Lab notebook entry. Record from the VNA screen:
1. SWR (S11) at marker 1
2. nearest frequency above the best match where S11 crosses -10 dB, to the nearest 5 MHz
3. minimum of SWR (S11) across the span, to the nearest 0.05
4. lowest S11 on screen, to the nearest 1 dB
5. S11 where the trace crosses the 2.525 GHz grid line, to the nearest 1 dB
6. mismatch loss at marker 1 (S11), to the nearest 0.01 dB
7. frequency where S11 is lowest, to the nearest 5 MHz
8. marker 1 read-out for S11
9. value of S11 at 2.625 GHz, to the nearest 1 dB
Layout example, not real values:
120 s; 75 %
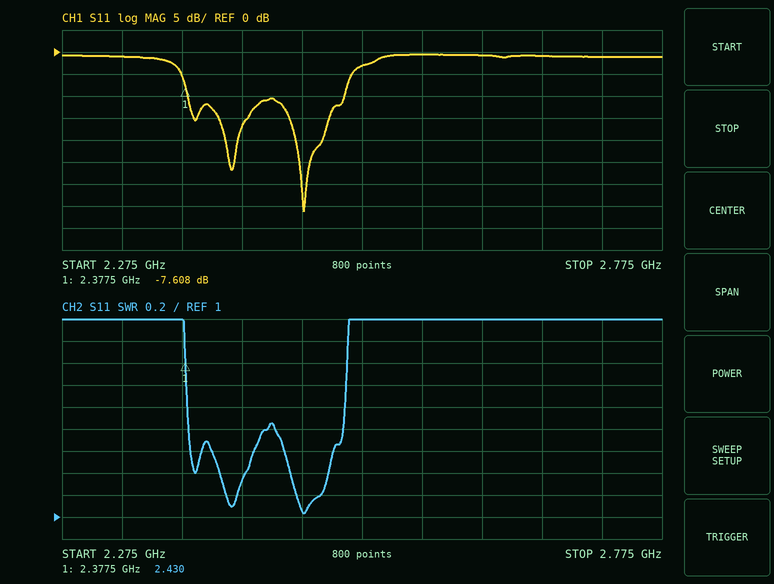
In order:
2.430; 2.510 GHz; 1.05; -36 dB; -3 dB; 0.83 dB; 2.475 GHz; -7.608 dB; -1 dB
